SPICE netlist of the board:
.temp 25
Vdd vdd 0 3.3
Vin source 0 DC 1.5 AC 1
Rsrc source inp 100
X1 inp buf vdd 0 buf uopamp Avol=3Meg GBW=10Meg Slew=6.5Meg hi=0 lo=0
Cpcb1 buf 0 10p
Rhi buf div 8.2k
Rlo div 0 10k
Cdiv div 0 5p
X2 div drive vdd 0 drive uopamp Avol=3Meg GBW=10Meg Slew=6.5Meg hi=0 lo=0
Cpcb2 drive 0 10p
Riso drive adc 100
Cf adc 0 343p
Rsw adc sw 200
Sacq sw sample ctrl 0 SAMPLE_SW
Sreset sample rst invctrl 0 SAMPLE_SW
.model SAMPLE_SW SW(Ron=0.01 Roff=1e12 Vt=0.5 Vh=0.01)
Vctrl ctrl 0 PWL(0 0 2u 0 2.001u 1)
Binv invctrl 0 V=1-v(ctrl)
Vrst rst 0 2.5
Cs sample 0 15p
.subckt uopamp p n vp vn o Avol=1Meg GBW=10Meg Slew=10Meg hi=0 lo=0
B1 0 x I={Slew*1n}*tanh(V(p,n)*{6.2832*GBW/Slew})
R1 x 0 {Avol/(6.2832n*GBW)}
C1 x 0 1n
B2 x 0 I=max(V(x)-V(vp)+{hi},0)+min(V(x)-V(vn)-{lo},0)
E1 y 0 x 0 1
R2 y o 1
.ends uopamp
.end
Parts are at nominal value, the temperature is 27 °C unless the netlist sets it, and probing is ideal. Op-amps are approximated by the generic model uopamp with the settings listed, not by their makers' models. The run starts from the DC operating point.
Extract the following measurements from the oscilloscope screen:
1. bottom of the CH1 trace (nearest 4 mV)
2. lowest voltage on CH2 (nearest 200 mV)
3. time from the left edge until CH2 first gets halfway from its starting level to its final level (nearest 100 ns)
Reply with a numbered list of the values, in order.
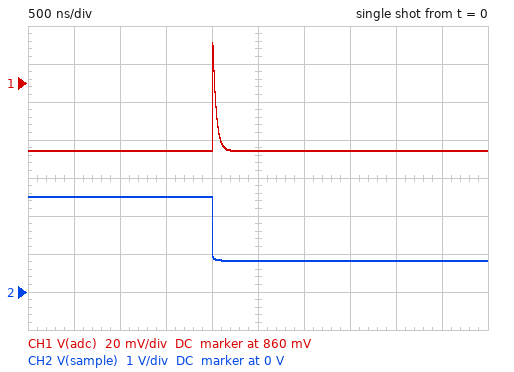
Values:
1. 824 mV
2. 800 mV
3. 2.0 µs
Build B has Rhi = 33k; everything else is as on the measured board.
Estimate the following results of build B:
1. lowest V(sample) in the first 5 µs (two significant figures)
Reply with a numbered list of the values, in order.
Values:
1. 350 mV
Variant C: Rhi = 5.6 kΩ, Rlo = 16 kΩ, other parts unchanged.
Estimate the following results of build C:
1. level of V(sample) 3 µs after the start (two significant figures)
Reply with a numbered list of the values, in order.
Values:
1. 1.1 V
